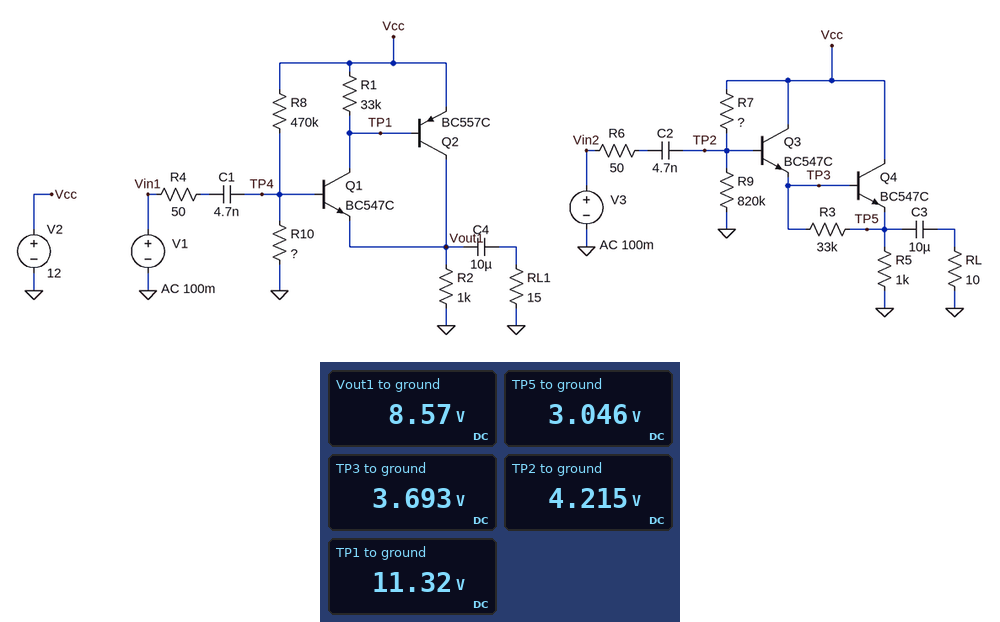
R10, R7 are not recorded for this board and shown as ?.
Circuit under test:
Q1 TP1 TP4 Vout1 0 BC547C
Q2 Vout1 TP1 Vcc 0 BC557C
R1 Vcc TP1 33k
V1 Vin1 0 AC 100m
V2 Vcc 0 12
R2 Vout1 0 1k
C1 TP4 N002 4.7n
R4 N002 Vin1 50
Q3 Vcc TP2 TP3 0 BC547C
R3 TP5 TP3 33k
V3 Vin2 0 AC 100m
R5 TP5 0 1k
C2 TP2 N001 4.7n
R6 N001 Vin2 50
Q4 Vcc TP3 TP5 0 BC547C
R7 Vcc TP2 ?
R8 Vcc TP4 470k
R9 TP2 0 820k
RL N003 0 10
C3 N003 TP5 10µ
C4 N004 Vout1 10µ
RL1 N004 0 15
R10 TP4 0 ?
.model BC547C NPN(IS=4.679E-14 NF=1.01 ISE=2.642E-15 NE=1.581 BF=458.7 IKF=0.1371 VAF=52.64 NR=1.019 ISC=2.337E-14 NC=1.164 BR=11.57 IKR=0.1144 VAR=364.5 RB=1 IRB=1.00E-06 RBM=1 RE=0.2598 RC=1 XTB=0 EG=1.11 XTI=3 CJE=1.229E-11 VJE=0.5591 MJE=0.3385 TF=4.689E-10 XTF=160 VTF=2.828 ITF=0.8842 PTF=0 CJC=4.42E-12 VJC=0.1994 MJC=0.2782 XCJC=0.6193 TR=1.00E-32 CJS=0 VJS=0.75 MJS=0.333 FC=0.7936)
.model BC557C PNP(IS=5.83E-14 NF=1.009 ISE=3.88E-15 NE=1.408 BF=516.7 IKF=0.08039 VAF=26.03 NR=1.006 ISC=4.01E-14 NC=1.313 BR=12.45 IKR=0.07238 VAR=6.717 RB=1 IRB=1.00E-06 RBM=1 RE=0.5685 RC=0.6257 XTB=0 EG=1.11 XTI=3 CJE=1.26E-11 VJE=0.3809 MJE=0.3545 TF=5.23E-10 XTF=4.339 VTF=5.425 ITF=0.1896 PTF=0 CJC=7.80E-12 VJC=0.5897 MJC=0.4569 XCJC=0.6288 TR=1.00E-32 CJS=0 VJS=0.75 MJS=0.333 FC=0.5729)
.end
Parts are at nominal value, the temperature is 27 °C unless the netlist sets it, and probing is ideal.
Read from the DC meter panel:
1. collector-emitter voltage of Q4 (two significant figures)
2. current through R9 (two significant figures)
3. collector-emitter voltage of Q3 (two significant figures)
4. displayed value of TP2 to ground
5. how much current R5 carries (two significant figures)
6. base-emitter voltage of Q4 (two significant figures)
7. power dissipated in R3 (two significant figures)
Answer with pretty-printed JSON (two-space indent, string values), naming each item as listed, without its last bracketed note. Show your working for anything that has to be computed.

{
  "collector-emitter voltage of Q4": "12 V - 3.046 V = 9.0 V",
  "current through R9": "(4.215 V) / 820 kΩ = 5.1 µA",
  "collector-emitter voltage of Q3": "12 V - 3.693 V = 8.3 V",
  "displayed value of TP2 to ground": "4.215 V",
  "how much current R5 carries": "(3.046 V) / 1 kΩ = 3.0 mA",
  "base-emitter voltage of Q4": "3.693 V - 3.046 V = 650 mV",
  "power dissipated in R3": "(3.693 V - 3.046 V)^2 / 33 kΩ = 13 µW"
}
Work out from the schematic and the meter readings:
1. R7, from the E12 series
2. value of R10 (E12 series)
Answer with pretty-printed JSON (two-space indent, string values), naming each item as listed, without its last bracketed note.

{
  "R7, from the E12 series": "1.5 MΩ",
  "value of R10": "1.5 MΩ"
}
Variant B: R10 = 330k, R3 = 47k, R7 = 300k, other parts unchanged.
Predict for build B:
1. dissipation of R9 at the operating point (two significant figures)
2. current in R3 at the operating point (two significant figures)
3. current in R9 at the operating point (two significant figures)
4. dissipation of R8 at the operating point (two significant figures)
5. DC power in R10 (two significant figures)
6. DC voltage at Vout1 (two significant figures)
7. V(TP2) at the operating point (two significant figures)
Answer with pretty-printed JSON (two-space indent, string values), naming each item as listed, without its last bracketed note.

{
  "dissipation of R9 at the operating point": "94 µW",
  "current in R3 at the operating point": "14 µA",
  "current in R9 at the operating point": "11 µA",
  "dissipation of R8 at the operating point": "110 µW",
  "DC power in R10": "74 µW",
  "DC voltage at Vout1": "4.4 V",
  "V(TP2) at the operating point": "8.8 V"
}
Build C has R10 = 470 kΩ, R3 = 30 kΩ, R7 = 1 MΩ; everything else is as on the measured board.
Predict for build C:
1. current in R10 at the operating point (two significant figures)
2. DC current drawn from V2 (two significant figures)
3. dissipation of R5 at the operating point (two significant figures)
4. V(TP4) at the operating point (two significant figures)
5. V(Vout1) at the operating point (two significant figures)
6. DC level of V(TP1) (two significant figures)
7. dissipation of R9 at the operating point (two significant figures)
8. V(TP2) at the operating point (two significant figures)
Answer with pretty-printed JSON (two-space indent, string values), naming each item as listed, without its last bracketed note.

{
  "current in R10 at the operating point": "13 µA",
  "DC current drawn from V2": "9.7 mA",
  "dissipation of R5 at the operating point": "18 mW",
  "V(TP4) at the operating point": "6.0 V",
  "V(Vout1) at the operating point": "5.5 V",
  "DC level of V(TP1)": "11 V",
  "dissipation of R9 at the operating point": "35 µW",
  "V(TP2) at the operating point": "5.4 V"
}
